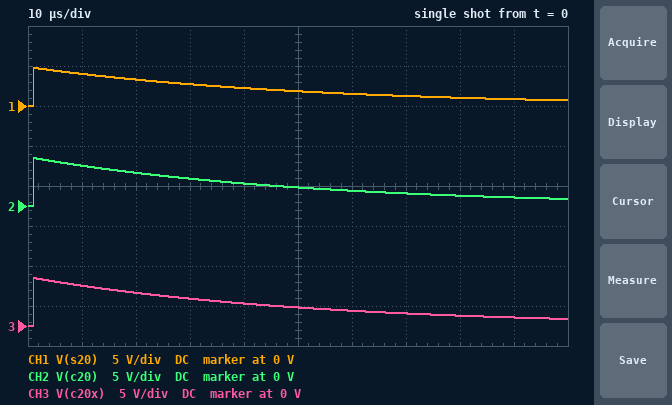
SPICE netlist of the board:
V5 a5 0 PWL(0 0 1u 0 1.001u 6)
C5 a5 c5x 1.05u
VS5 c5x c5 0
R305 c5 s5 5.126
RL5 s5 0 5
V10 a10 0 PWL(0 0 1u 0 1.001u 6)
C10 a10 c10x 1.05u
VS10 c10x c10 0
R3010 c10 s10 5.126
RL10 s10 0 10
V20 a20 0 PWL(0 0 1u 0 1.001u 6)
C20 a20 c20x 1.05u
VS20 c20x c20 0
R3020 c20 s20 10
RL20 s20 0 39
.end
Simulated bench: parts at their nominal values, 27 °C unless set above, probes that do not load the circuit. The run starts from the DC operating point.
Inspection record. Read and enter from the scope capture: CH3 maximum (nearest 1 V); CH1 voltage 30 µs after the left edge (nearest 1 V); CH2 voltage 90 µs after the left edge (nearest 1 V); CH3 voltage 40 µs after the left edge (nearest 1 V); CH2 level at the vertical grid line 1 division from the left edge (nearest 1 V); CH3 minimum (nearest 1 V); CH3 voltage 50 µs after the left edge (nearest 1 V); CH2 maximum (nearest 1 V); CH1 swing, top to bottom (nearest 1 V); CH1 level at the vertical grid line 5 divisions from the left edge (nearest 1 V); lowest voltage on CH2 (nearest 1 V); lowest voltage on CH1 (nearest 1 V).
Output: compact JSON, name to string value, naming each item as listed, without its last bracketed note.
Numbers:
{"CH3 maximum": "6 V", "CH1 voltage 30 µs after the left edge": "3 V", "CH2 voltage 90 µs after the left edge": "1 V", "CH3 voltage 40 µs after the left edge": "3 V", "CH2 level at the vertical grid line 1 division from the left edge": "5 V", "CH3 minimum": "0 V", "CH3 voltage 50 µs after the left edge": "2 V", "CH2 maximum": "6 V", "CH1 swing, top to bottom": "5 V", "CH1 level at the vertical grid line 5 divisions from the left edge": "2 V", "lowest voltage on CH2": "0 V", "lowest voltage on CH1": "0 V"}
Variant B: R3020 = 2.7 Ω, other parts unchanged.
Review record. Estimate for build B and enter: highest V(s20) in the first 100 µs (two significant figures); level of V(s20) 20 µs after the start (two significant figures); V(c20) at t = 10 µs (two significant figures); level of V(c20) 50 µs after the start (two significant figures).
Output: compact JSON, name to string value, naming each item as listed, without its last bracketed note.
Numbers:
{"highest V(s20) in the first 100 µs": "5.6 V", "level of V(s20) 20 µs after the start": "3.6 V", "V(c20) at t = 10 µs": "4.9 V", "level of V(c20) 50 µs after the start": "2.0 V"}
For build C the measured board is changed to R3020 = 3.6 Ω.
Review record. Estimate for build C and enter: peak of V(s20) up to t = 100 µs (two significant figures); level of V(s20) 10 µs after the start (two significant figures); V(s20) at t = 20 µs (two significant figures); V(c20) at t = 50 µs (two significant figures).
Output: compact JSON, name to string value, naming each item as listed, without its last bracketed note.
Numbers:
{"peak of V(s20) up to t = 100 µs": "5.5 V", "level of V(s20) 10 µs after the start": "4.5 V", "V(s20) at t = 20 µs": "3.6 V", "V(c20) at t = 50 µs": "2.0 V"}
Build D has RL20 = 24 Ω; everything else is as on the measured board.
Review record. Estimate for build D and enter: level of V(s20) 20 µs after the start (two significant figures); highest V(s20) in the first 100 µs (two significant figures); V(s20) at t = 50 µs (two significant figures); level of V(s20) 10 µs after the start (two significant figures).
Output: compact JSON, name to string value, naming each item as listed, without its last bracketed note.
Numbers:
{"level of V(s20) 20 µs after the start": "2.5 V", "highest V(s20) in the first 100 µs": "4.2 V", "V(s20) at t = 50 µs": "1.1 V", "level of V(s20) 10 µs after the start": "3.3 V"}
